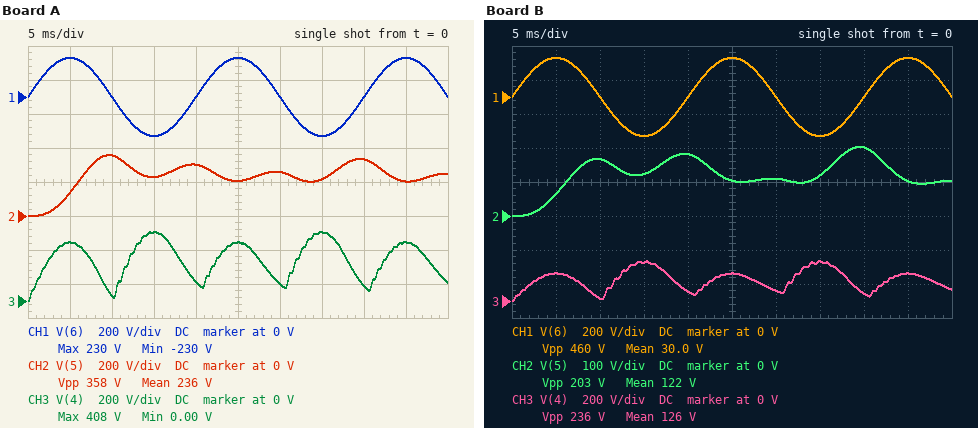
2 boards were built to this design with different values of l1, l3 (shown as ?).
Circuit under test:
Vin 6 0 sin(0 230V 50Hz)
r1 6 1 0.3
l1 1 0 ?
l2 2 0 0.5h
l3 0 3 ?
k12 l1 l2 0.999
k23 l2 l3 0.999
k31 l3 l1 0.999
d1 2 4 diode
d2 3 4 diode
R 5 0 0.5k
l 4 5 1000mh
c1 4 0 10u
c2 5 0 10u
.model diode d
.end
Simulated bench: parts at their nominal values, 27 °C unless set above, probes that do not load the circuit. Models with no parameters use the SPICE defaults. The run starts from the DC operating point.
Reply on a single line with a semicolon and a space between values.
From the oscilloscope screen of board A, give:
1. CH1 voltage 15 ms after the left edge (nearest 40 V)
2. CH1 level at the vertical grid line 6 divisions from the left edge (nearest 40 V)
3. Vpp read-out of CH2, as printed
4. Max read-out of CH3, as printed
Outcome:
-240 V; 0 V; 358 V; 408 V
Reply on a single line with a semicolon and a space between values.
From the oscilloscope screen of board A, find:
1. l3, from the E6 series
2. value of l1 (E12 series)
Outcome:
680 mH; 220 mH
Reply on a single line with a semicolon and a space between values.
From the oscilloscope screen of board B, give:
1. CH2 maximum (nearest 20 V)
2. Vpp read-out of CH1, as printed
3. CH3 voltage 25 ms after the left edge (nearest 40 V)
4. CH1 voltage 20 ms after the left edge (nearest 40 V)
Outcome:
200 V; 460 V; 160 V; 0 V
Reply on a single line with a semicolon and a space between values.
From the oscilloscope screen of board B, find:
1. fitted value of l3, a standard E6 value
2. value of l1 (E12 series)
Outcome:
1 H; 1 H
